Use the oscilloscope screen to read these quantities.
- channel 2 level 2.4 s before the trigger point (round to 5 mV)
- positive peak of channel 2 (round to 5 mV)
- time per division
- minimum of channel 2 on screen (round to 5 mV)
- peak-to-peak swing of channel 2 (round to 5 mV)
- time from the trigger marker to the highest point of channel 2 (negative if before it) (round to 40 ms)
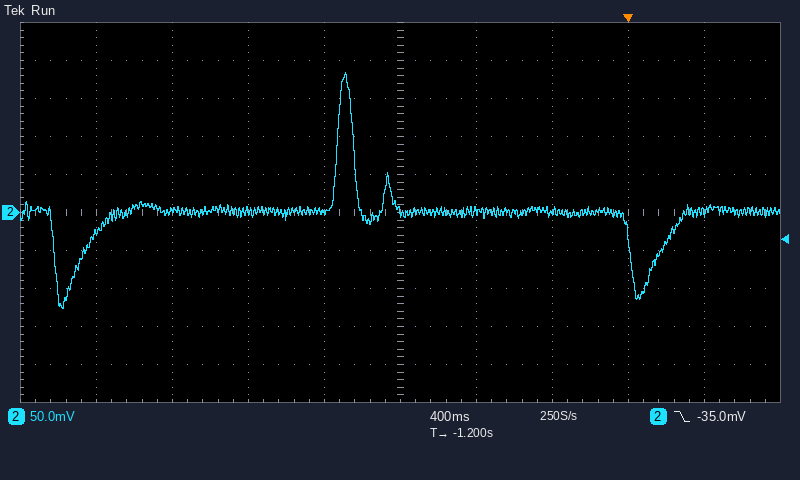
0 mV
185 mV
400 ms
-125 mV
310 mV
-1.48 s
